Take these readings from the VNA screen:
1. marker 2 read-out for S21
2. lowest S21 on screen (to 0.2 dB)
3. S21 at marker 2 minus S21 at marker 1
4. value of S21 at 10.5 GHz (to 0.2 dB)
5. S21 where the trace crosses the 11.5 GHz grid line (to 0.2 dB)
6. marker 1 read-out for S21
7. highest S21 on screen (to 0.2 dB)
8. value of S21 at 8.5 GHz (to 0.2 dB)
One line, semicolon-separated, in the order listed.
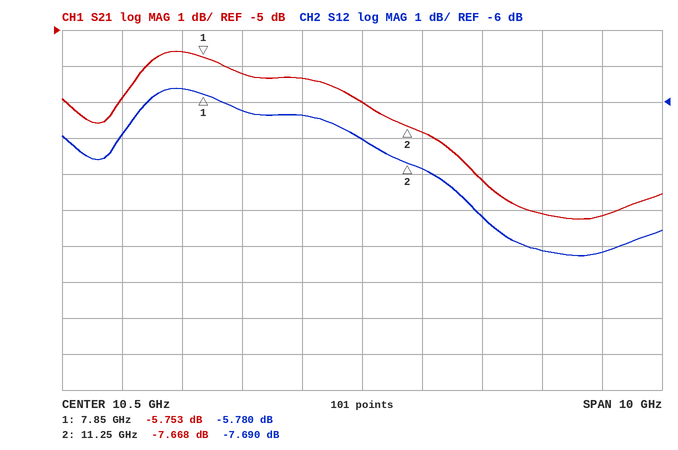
-7.668 dB; -10.2 dB; -1.915 dB; -7.0 dB; -7.8 dB; -5.753 dB; -5.6 dB; -6.2 dB
